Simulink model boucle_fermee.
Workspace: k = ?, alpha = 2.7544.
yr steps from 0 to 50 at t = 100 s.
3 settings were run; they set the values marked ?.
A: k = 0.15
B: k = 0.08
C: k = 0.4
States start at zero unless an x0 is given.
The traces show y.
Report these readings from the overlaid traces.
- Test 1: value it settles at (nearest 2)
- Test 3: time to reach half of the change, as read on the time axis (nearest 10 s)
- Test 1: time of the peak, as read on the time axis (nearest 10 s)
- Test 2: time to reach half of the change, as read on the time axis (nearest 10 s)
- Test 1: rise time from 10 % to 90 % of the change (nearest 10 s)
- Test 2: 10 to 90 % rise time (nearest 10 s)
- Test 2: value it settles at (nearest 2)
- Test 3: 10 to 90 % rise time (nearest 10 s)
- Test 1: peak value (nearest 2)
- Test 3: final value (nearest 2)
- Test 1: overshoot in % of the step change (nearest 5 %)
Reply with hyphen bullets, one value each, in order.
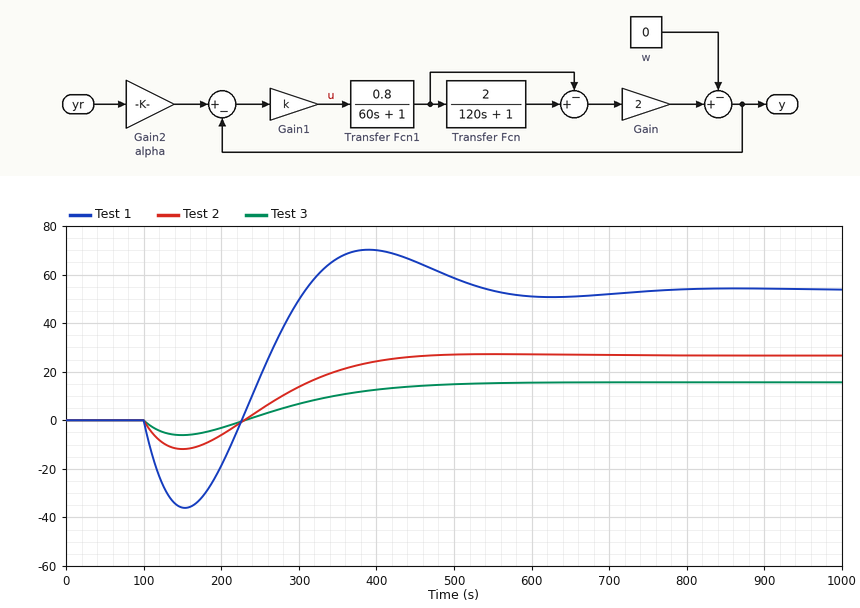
- 54
- 310 s
- 390 s
- 300 s
- 60 s
- 150 s
- 26
- 210 s
- 70
- 16
- 30 %
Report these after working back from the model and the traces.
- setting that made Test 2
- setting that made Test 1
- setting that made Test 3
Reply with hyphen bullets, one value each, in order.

- A
- C
- B
